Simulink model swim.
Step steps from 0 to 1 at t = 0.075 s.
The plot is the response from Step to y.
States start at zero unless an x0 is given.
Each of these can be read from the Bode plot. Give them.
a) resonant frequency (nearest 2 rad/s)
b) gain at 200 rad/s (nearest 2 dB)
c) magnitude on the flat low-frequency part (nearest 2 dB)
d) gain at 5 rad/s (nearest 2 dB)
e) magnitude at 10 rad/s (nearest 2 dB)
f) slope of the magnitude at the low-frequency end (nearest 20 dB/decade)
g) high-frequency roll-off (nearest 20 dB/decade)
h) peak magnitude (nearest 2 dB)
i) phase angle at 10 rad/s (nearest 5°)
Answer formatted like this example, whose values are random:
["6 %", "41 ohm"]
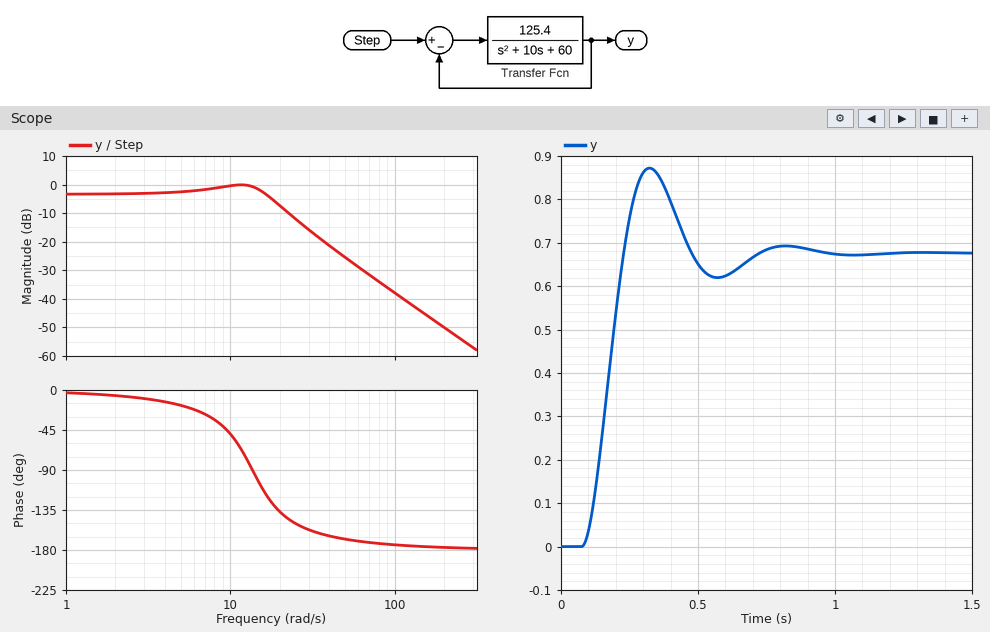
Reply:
["12 rad/s", "-50 dB", "-4 dB", "-2 dB", "0 dB", "0 dB/decade", "-40 dB/decade", "0 dB", "-50°"]
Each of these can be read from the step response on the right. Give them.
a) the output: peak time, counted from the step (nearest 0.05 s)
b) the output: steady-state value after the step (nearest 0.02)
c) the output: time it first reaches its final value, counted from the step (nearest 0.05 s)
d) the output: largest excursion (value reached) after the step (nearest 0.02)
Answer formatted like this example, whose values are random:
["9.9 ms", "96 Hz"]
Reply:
["0.25 s", "0.68", "0.15 s", "0.88"]
